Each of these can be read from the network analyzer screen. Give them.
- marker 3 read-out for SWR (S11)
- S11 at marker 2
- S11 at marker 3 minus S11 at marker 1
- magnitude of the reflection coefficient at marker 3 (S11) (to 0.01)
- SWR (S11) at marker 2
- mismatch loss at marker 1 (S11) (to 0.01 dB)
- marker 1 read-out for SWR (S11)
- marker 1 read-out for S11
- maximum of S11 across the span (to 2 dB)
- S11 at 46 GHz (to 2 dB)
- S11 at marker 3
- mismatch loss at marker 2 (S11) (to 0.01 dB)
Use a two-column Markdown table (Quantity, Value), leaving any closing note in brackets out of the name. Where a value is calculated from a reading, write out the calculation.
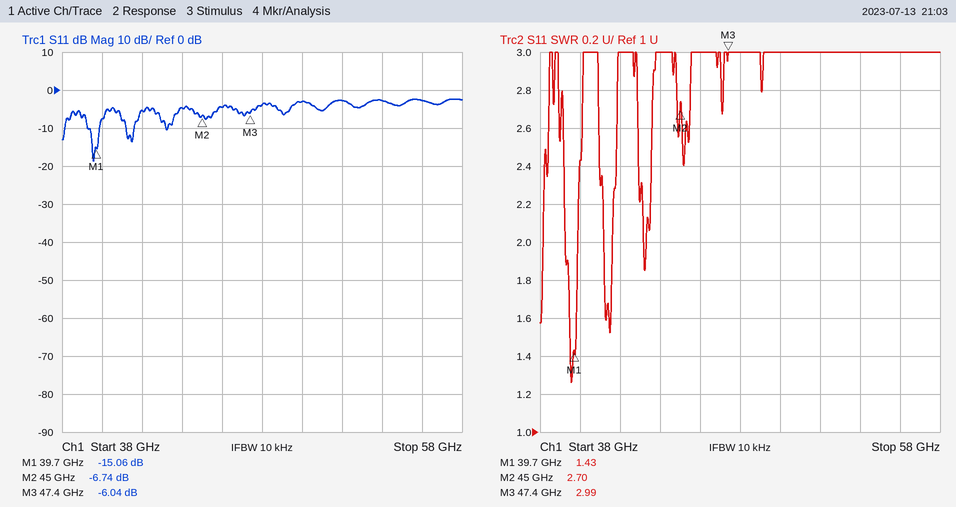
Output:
| Quantity | Value |
|---|---|
| marker 3 read-out for SWR | 2.99 |
| S11 at marker 2 | -6.74 dB |
| S11 at marker 3 minus S11 at marker 1 | -6.04 − (-15.06) = 9.02 dB |
| magnitude of the reflection coefficient at marker 3 (S11) | 10^(-6.04/20) ≈ 0.50 |
| SWR (S11) at marker 2 | 2.70 |
| mismatch loss at marker 1 (S11) | −10 log10(1 − 10^(-15.06/10)) ≈ 0.14 dB |
| marker 1 read-out for SWR | 1.43 |
| marker 1 read-out for S11 | -15.06 dB |
| maximum of S11 across the span | -2 dB |
| S11 at 46 GHz | -4 dB |
| S11 at marker 3 | -6.04 dB |
| mismatch loss at marker 2 (S11) | −10 log10(1 − 10^(-6.74/10)) ≈ 1.03 dB |
